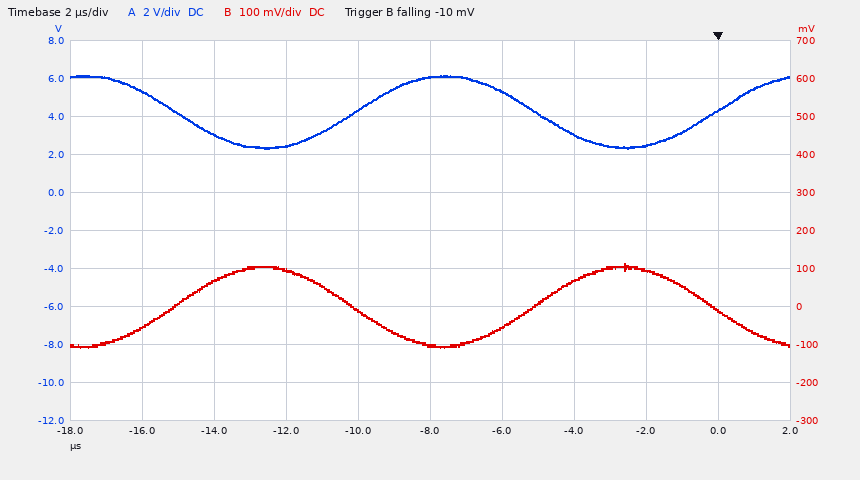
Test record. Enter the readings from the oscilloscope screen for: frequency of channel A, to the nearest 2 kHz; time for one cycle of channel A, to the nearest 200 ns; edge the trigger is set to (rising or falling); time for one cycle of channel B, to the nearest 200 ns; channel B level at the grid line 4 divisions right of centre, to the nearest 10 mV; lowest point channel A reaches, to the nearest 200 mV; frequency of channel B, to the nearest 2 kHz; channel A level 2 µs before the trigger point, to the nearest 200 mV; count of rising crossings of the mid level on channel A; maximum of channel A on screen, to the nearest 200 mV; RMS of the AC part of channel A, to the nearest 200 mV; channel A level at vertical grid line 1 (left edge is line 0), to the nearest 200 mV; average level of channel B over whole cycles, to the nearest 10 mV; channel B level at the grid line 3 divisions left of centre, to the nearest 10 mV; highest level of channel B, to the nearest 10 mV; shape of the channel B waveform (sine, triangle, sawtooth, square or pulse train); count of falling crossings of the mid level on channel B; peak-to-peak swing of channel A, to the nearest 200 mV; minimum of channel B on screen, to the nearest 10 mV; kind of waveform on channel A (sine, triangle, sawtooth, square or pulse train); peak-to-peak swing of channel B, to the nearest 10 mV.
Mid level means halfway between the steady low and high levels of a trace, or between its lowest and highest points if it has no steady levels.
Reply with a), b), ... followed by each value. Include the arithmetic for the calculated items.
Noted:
a) 1 / 10.0 µs ≈ 100 kHz
b) 10.0 µs
c) falling
d) 10.0 µs
e) -10 mV
f) 2.4 V
g) 1 / 10.0 µs ≈ 100 kHz
h) 2.4 V
i) 2
j) 6.2 V
k) 3.8 V / (2√2) ≈ 1.34 V, so 1.4 V to the nearest 200 mV
l) 5.4 V
m) (110 mV + (-110 mV)) / 2 ≈ 0 mV
n) 70 mV
o) 110 mV
p) sine
q) 2
r) 6.2 V − (2.4 V) = 3.8 V
s) -110 mV
t) sine
u) 110 mV − (-110 mV) = 220 mV
